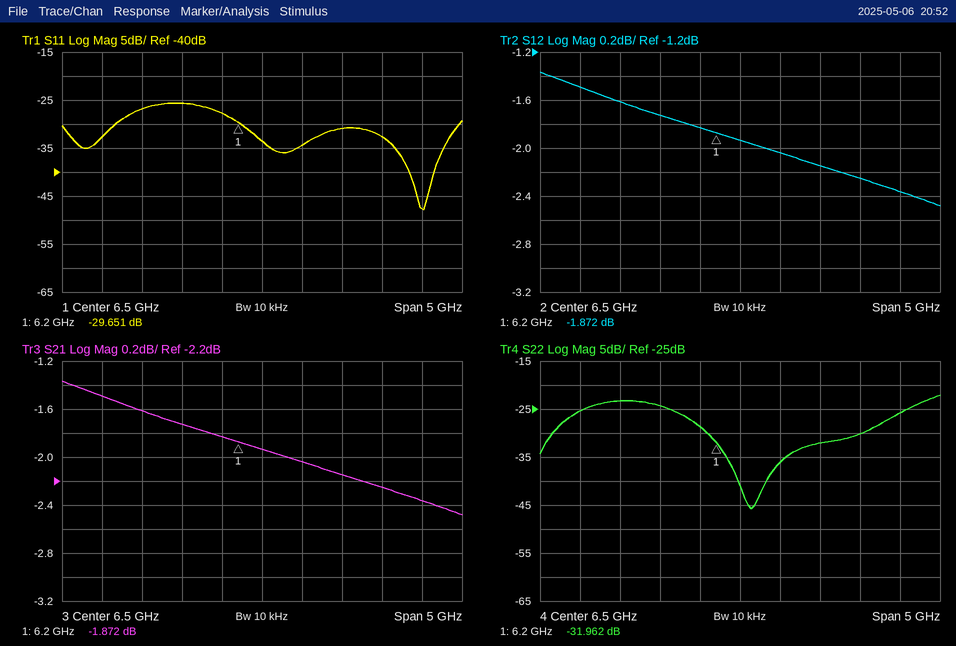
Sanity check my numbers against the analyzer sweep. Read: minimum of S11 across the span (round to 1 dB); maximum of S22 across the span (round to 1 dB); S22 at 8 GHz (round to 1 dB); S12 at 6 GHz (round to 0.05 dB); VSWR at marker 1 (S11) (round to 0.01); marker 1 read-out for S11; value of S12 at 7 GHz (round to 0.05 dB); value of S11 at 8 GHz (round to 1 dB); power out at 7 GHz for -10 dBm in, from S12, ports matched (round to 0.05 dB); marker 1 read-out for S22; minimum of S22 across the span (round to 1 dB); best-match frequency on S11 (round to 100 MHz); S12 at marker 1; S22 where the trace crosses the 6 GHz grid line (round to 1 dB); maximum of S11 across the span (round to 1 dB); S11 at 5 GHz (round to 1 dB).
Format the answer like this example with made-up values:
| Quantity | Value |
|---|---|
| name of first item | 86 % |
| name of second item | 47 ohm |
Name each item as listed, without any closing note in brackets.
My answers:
| Quantity | Value |
|---|---|
| minimum of S11 across the span | -48 dB |
| maximum of S22 across the span | -22 dB |
| S22 at 8 GHz | -30 dB |
| S12 at 6 GHz | -1.85 dB |
| VSWR at marker 1 (S11) | 1.07 |
| marker 1 read-out for S11 | -29.651 dB |
| value of S12 at 7 GHz | -2.05 dB |
| value of S11 at 8 GHz | -33 dB |
| power out at 7 GHz for -10 dBm in, from S12, ports matched | -12.05 dBm |
| marker 1 read-out for S22 | -31.962 dB |
| minimum of S22 across the span | -46 dB |
| best-match frequency on S11 | 8.5 GHz |
| S12 at marker 1 | -1.872 dB |
| S22 where the trace crosses the 6 GHz grid line | -29 dB |
| maximum of S11 across the span | -26 dB |
| S11 at 5 GHz | -27 dB |
